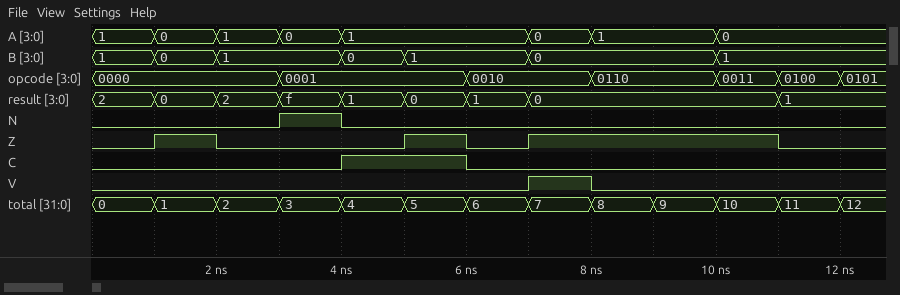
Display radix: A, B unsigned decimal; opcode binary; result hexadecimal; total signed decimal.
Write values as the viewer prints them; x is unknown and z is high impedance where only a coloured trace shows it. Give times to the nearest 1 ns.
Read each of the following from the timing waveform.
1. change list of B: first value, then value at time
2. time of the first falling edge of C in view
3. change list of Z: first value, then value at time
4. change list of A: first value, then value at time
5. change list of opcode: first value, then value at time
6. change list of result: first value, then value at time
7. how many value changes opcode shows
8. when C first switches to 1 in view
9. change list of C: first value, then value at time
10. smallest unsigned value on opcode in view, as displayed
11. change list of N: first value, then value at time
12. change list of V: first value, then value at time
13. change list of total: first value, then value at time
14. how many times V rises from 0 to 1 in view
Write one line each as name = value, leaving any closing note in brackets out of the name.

change list of B: first value, then value at time = 1, 0 at 1 ns, 1 at 2 ns, 0 at 4 ns, 1 at 5 ns, 0 at 7 ns, 1 at 10 ns
time of the first falling edge of C in view = 6 ns
change list of Z: first value, then value at time = 0, 1 at 1 ns, 0 at 2 ns, 1 at 5 ns, 0 at 6 ns, 1 at 7 ns, 0 at 11 ns
change list of A: first value, then value at time = 1, 0 at 1 ns, 1 at 2 ns, 0 at 3 ns, 1 at 4 ns, 0 at 7 ns, 1 at 8 ns, 0 at 10 ns
change list of opcode: first value, then value at time = 0000, 0001 at 3 ns, 0010 at 6 ns, 0110 at 8 ns, 0011 at 10 ns, 0100 at 11 ns, 0101 at 12 ns
change list of result: first value, then value at time = 2, 0 at 1 ns, 2 at 2 ns, f at 3 ns, 1 at 4 ns, 0 at 5 ns, 1 at 6 ns, 0 at 7 ns, 1 at 11 ns
how many value changes opcode shows = 6
when C first switches to 1 in view = 4 ns
change list of C: first value, then value at time = 0, 1 at 4 ns, 0 at 6 ns
smallest unsigned value on opcode in view, as displayed = 0000
change list of N: first value, then value at time = 0, 1 at 3 ns, 0 at 4 ns
change list of V: first value, then value at time = 0, 1 at 7 ns, 0 at 8 ns
change list of total: first value, then value at time = 0, 1 at 1 ns, 2 at 2 ns, 3 at 3 ns, 4 at 4 ns, 5 at 5 ns, 6 at 6 ns, 7 at 7 ns, 8 at 8 ns, 9 at 9 ns, 10 at 10 ns, 11 at 11 ns, 12 at 12 ns
how many times V rises from 0 to 1 in view = 1
